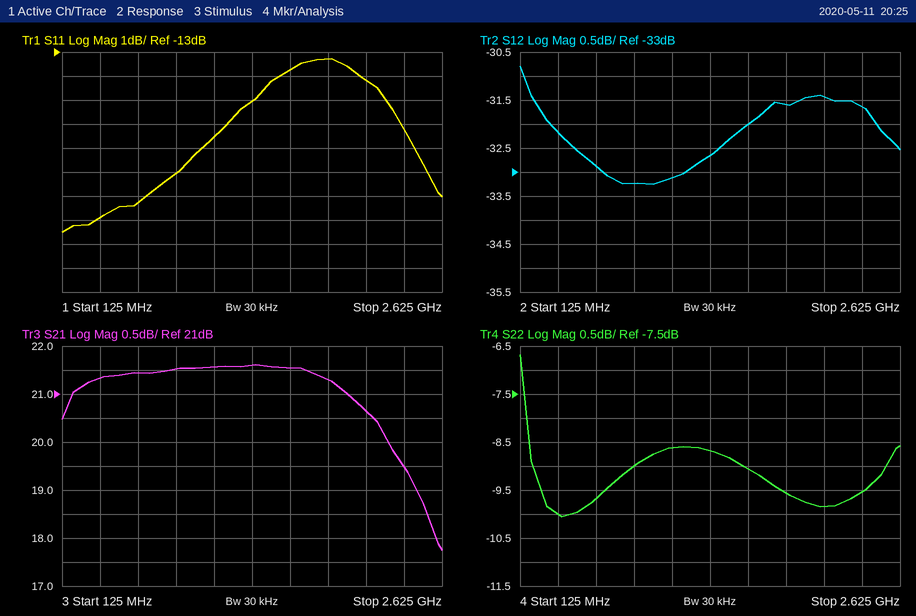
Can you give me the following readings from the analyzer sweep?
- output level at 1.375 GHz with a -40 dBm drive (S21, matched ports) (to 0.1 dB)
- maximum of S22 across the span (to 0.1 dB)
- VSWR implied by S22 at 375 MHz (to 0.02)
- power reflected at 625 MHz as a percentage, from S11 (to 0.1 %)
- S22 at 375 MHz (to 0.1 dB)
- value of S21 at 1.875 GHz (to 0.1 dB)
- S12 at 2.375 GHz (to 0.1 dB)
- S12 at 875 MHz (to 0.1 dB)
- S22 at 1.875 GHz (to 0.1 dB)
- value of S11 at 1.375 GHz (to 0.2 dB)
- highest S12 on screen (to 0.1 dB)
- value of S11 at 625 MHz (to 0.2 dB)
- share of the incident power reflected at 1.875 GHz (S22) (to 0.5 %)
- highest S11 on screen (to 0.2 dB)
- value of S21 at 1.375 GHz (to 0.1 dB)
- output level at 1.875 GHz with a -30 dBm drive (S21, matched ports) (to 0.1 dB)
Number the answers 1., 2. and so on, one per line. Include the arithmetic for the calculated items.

1. -40 dBm + (21.6 dB) = -18.4 dBm
2. -6.7 dB
3. |Γ| = 10^(-10/20) = 0.3162; VSWR = (1 + 0.3162)/(1 − 0.3162) ≈ 1.92
4. 10^(-19.2/10) ≈ 1.2 %
5. -10.0 dB
6. 21.3 dB
7. -31.6 dB
8. -33.2 dB
9. -9.6 dB
10. -15.0 dB
11. -30.8 dB
12. -19.2 dB
13. 10^(-9.6/10) ≈ 11.0 %
14. -13.2 dB
15. 21.6 dB
16. -30 dBm + (21.3 dB) = -8.7 dBm
